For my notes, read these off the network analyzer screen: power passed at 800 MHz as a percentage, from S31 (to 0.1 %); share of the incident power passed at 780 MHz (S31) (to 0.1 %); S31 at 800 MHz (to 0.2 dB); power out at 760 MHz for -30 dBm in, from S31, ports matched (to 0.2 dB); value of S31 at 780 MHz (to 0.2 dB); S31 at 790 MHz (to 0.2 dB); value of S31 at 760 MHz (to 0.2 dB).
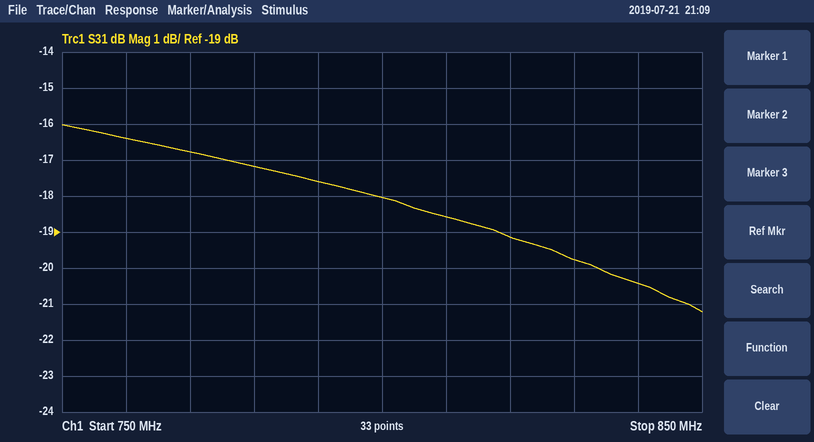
1.6 %
1.9 %
-18.0 dB
-46.4 dBm
-17.2 dB
-17.6 dB
-16.4 dB
